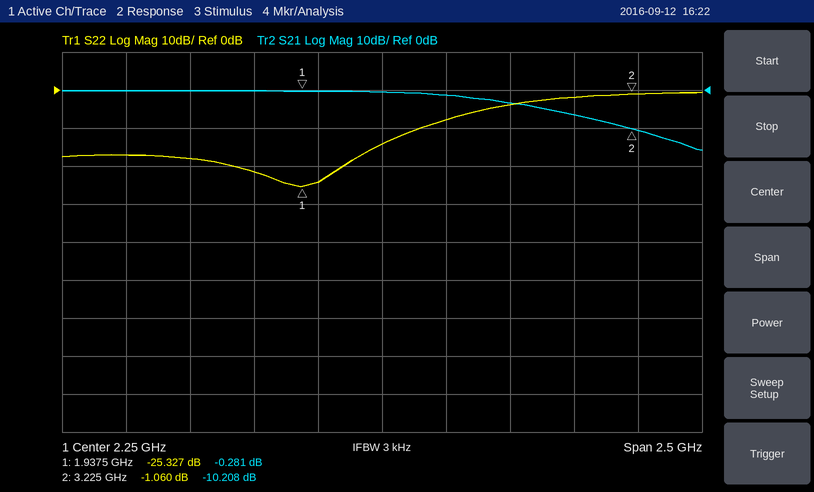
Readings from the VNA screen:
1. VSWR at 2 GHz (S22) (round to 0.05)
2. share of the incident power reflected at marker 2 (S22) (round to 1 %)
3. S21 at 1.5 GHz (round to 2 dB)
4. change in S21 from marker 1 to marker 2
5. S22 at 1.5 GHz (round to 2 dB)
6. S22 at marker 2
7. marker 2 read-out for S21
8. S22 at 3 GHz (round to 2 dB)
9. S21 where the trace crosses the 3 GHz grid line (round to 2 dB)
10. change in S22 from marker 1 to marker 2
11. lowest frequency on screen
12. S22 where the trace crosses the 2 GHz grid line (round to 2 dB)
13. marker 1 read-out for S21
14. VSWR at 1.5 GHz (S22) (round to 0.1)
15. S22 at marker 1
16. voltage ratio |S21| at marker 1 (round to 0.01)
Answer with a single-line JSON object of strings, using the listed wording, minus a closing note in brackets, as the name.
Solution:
{"VSWR at 2 GHz (S22)": "1.15", "share of the incident power reflected at marker 2 (S22)": "78 %", "S21 at 1.5 GHz": "0 dB", "change in S21 from marker 1 to marker 2": "-9.927 dB", "S22 at 1.5 GHz": "-18 dB", "S22 at marker 2": "-1.060 dB", "marker 2 read-out for S21": "-10.208 dB", "S22 at 3 GHz": "-2 dB", "S21 where the trace crosses the 3 GHz grid line": "-6 dB", "change in S22 from marker 1 to marker 2": "24.267 dB", "lowest frequency on screen": "1 GHz", "S22 where the trace crosses the 2 GHz grid line": "-24 dB", "marker 1 read-out for S21": "-0.281 dB", "VSWR at 1.5 GHz (S22)": "1.3", "S22 at marker 1": "-25.327 dB", "voltage ratio |S21| at marker 1": "0.97"}
